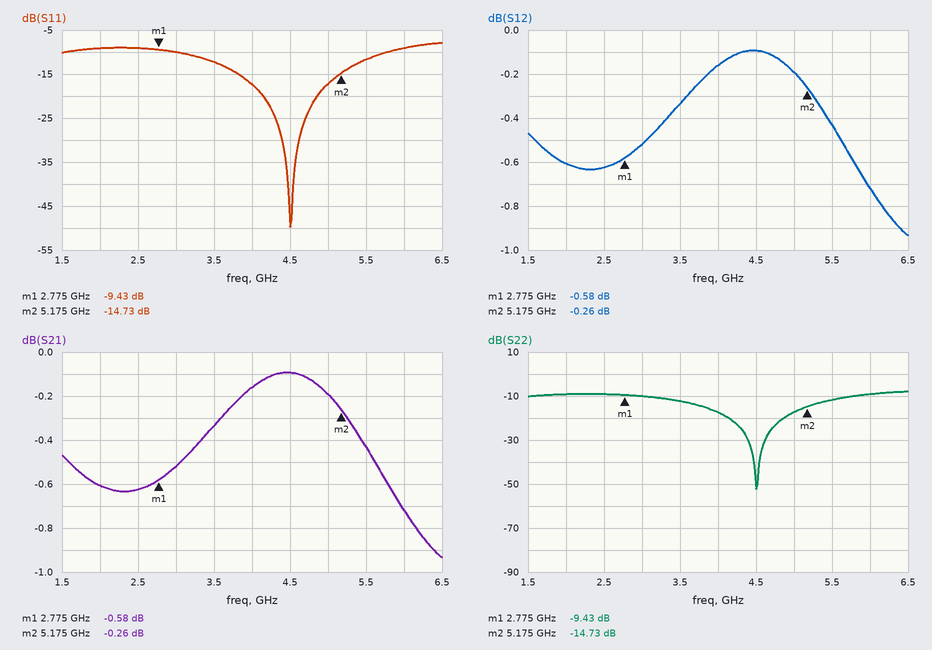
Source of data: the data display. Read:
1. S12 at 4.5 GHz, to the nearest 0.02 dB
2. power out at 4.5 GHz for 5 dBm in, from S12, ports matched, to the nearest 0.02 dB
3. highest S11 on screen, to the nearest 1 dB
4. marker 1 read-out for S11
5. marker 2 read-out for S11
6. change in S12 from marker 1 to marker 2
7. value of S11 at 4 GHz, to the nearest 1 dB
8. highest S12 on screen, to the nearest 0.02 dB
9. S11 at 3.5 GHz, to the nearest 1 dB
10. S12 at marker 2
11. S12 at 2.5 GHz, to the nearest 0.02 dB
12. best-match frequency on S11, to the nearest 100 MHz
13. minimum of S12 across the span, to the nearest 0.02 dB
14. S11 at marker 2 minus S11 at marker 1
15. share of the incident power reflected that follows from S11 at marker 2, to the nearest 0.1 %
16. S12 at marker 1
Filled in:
-0.10 dB
4.90 dBm
-8 dB
-9.43 dB
-14.73 dB
0.32 dB
-17 dB
-0.10 dB
-12 dB
-0.26 dB
-0.62 dB
4.5 GHz
-0.94 dB
-5.30 dB
3.4 %
-0.58 dB
